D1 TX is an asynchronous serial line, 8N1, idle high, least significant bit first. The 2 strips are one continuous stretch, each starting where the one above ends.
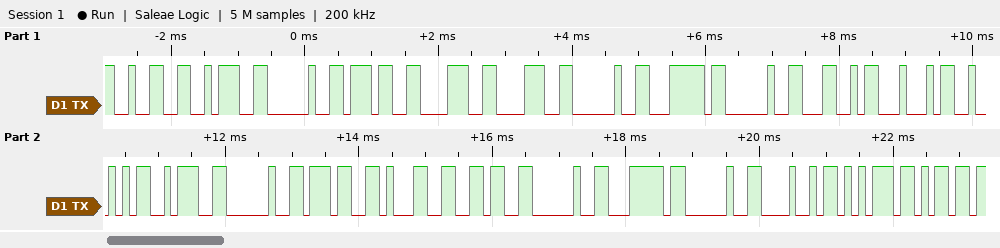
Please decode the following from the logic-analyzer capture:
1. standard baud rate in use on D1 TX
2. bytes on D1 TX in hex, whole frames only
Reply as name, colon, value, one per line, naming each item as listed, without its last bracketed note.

standard baud rate in use on D1 TX: 9600 baud
bytes on D1 TX in hex, whole frames only: 32 3A 20 37 38 38 20 7C 20 4C 44 52 3A 20 37 31 36 20 7C 20 48 75 6D
